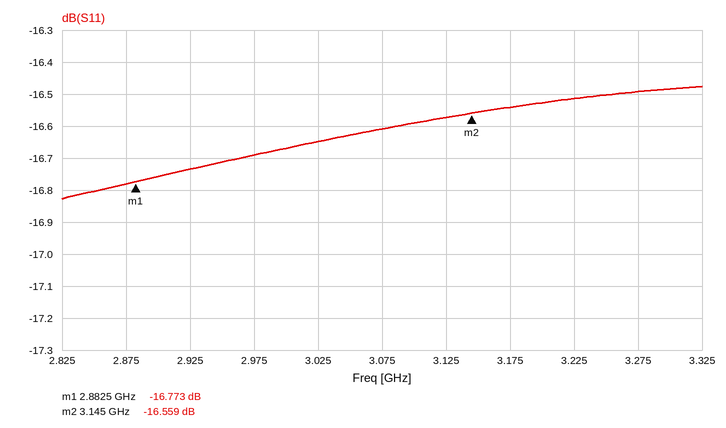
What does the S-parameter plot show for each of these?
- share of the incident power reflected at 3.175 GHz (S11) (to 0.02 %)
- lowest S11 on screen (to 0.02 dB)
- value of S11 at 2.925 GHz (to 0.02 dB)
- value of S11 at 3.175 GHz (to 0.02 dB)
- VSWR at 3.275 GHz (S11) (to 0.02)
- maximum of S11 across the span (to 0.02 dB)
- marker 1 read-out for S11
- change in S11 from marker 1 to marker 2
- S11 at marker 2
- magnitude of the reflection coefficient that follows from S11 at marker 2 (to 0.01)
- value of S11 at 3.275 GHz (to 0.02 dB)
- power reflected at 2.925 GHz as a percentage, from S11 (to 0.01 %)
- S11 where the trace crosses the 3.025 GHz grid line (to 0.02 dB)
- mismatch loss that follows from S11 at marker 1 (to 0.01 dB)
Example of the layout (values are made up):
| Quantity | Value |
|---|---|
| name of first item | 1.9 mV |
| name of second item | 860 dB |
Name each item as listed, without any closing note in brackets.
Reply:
| Quantity | Value |
|---|---|
| share of the incident power reflected at 3.175 GHz (S11) | 2.22 % |
| lowest S11 on screen | -16.82 dB |
| value of S11 at 2.925 GHz | -16.74 dB |
| value of S11 at 3.175 GHz | -16.54 dB |
| VSWR at 3.275 GHz (S11) | 1.36 |
| maximum of S11 across the span | -16.48 dB |
| marker 1 read-out for S11 | -16.773 dB |
| change in S11 from marker 1 to marker 2 | 0.214 dB |
| S11 at marker 2 | -16.559 dB |
| magnitude of the reflection coefficient that follows from S11 at marker 2 | 0.15 |
| value of S11 at 3.275 GHz | -16.50 dB |
| power reflected at 2.925 GHz as a percentage, from S11 | 2.12 % |
| S11 where the trace crosses the 3.025 GHz grid line | -16.64 dB |
| mismatch loss that follows from S11 at marker 1 | 0.09 dB |
